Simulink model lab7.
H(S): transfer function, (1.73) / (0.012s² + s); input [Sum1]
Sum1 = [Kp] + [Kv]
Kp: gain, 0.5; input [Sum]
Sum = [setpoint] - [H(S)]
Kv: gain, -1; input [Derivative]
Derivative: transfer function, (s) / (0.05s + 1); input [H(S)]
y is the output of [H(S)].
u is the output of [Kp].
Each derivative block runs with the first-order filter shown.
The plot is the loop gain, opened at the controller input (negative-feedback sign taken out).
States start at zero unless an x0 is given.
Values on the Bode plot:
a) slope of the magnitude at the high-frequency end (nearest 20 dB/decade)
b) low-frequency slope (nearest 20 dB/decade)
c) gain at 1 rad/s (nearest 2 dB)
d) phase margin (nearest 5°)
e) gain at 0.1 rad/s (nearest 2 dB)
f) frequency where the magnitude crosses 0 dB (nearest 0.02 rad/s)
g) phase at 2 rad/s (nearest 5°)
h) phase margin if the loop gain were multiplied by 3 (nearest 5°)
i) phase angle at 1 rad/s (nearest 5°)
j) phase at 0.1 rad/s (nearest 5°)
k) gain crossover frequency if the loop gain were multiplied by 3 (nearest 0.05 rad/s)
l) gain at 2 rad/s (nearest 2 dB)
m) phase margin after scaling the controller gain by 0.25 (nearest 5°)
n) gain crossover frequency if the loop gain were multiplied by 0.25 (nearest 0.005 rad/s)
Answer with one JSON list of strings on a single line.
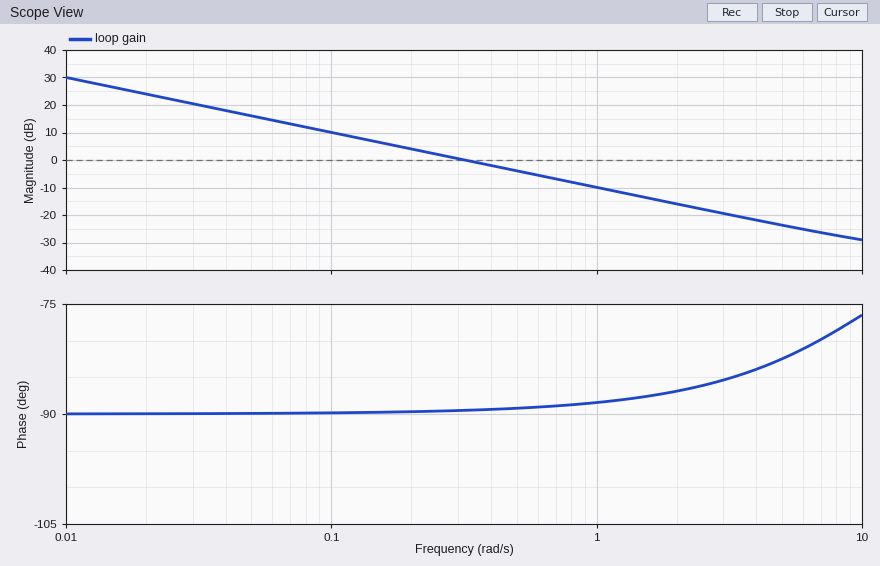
["-20 dB/decade", "-20 dB/decade", "-10 dB", "90°", "10 dB", "0.32 rad/s", "-85°", "90°", "-90°", "-90°", "0.95 rad/s", "-16 dB", "90°", "0.080 rad/s"]
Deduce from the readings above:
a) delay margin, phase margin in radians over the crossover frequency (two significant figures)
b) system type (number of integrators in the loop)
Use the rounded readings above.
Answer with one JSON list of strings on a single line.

["4.9 s", "1"]
